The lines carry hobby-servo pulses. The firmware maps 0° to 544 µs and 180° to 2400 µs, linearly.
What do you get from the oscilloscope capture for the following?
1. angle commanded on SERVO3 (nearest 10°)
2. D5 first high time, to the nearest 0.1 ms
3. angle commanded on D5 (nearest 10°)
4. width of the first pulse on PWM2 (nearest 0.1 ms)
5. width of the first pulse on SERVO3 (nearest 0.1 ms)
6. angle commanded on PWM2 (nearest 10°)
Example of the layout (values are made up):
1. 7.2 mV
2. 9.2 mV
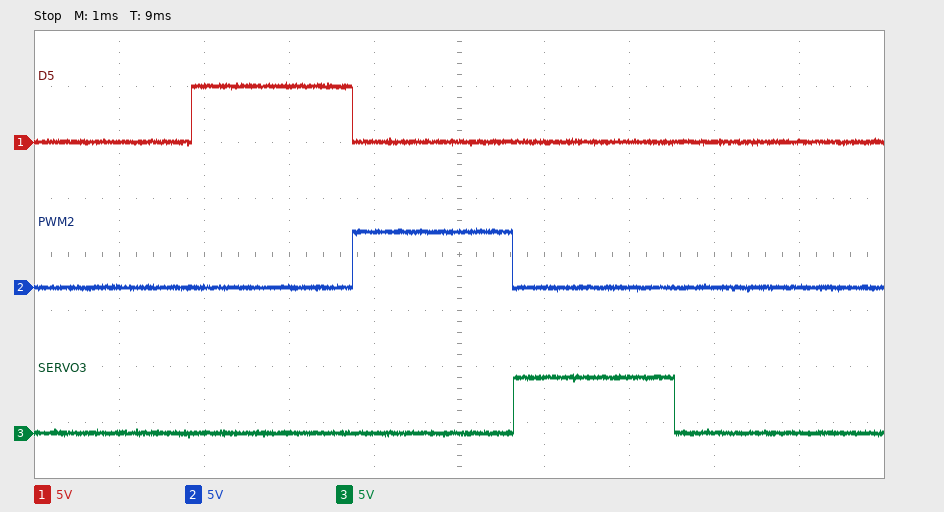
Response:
1. 130°
2. 1.9 ms
3. 130°
4. 1.9 ms
5. 1.9 ms
6. 130°
